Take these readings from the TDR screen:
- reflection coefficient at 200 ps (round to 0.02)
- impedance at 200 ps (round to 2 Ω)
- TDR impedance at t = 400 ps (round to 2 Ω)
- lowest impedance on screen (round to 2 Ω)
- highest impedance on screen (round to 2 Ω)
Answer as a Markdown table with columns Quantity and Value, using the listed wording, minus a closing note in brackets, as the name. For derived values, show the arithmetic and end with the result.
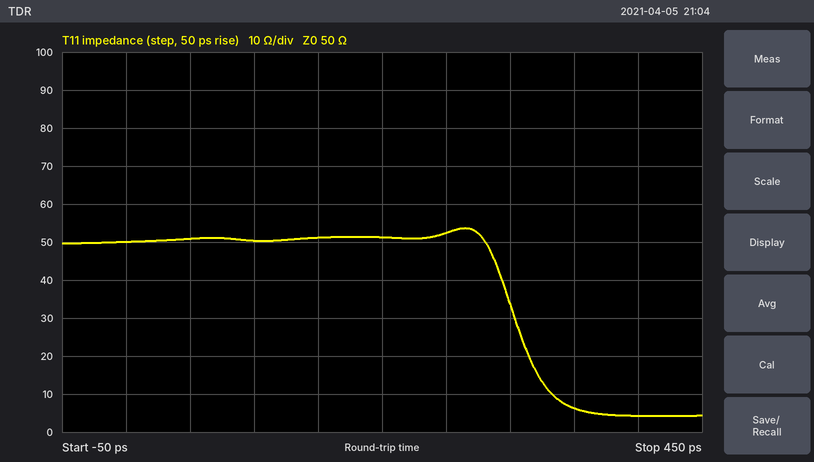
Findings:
| Quantity | Value |
|---|---|
| reflection coefficient at 200 ps | (52 − 50)/(52 + 50) ≈ +0.02 |
| impedance at 200 ps | 52 Ω |
| TDR impedance at t = 400 ps | 4 Ω |
| lowest impedance on screen | 4 Ω |
| highest impedance on screen | 54 Ω |
